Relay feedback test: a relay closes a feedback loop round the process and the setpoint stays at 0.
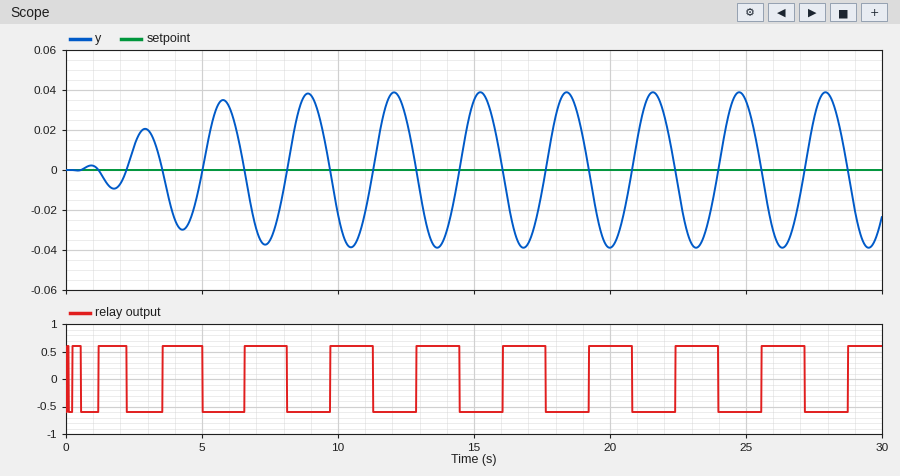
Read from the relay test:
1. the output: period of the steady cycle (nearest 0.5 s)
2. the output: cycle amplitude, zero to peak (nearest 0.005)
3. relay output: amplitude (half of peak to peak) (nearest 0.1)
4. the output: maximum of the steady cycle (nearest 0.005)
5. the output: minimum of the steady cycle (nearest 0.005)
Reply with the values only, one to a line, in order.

3.0 s
0.040
0.6
0.040
-0.040
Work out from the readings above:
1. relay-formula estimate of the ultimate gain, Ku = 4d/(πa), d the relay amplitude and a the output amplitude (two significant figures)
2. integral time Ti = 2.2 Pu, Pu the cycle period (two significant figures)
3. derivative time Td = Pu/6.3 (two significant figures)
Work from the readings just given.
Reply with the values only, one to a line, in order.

19
6.6 s
0.48 s
